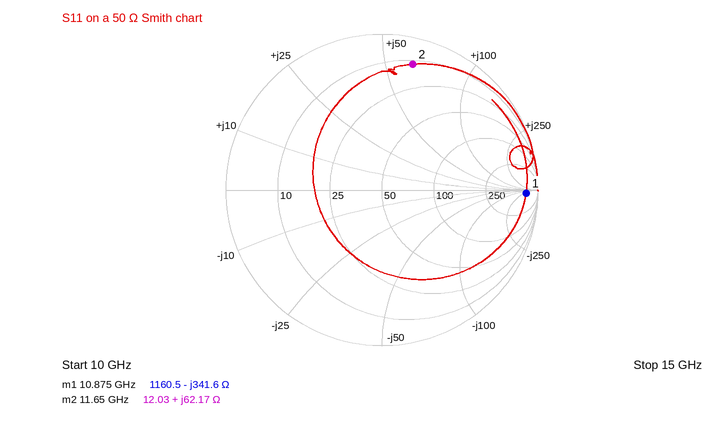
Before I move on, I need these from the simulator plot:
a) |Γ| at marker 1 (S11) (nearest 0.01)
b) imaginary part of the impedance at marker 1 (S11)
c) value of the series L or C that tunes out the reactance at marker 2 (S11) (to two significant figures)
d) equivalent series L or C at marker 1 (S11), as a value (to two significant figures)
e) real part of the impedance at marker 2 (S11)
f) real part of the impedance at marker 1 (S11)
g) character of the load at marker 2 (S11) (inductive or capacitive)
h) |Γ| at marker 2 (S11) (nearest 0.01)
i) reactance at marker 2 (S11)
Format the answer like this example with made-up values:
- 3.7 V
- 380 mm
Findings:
- 0.92
- -341.6 Ω
- 220 fF
- 43 fF
- 12.03 Ω
- 1160.5 Ω
- inductive
- 0.83
- +62.17 Ω
